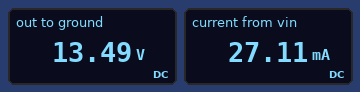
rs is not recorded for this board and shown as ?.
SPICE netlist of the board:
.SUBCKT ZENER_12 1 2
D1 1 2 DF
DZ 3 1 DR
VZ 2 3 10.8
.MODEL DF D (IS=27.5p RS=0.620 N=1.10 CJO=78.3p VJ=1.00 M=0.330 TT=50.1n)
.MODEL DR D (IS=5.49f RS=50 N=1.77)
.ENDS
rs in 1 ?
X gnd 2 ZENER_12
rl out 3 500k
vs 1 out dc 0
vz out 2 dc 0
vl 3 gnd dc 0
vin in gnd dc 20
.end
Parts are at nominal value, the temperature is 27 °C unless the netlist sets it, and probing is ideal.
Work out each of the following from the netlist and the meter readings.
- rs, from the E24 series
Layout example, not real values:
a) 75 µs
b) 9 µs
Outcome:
a) 240 Ω
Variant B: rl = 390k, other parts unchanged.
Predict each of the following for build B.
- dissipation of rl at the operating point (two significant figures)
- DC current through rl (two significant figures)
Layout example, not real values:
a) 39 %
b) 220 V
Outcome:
a) 470 µW
b) 35 µA
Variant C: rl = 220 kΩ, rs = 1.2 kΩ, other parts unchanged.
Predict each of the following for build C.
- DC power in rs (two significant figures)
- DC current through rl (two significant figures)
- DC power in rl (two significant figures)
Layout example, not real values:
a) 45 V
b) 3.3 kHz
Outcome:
a) 48 mW
b) 56 µA
c) 700 µW
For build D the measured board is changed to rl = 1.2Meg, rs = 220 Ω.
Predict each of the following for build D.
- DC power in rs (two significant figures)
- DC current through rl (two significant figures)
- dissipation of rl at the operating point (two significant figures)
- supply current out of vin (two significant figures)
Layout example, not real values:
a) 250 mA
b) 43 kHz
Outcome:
a) 190 mW
b) 11 µA
c) 150 µW
d) 29 mA
